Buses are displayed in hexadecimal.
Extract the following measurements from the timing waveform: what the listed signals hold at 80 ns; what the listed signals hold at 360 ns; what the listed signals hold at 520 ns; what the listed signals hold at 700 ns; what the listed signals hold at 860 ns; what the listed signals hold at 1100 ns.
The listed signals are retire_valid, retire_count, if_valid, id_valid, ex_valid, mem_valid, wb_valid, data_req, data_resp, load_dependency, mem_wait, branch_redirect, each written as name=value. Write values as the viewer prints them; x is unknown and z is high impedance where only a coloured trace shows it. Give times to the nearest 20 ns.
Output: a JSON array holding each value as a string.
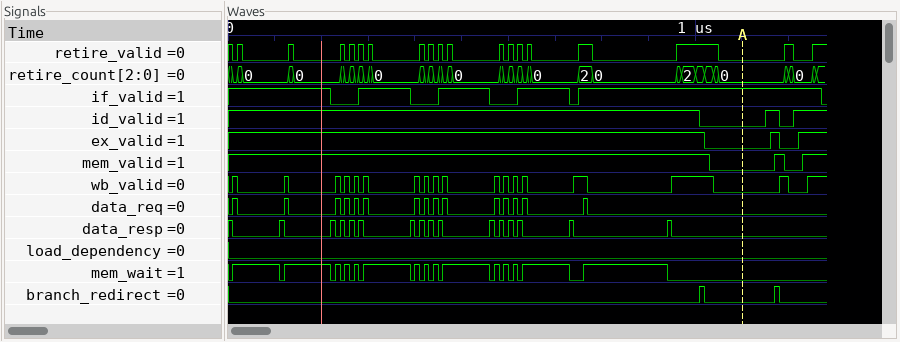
["retire_valid=0, retire_count=0, if_valid=1, id_valid=1, ex_valid=1, mem_valid=1, wb_valid=0, data_req=0, data_resp=0, load_dependency=0, mem_wait=1, branch_redirect=0", "retire_valid=0, retire_count=0, if_valid=1, id_valid=1, ex_valid=1, mem_valid=1, wb_valid=0, data_req=0, data_resp=0, load_dependency=0, mem_wait=1, branch_redirect=0", "retire_valid=0, retire_count=0, if_valid=1, id_valid=1, ex_valid=1, mem_valid=1, wb_valid=0, data_req=0, data_resp=0, load_dependency=0, mem_wait=1, branch_redirect=0", "retire_valid=0, retire_count=0, if_valid=1, id_valid=1, ex_valid=1, mem_valid=1, wb_valid=0, data_req=0, data_resp=0, load_dependency=0, mem_wait=1, branch_redirect=0", "retire_valid=0, retire_count=0, if_valid=1, id_valid=1, ex_valid=1, mem_valid=1, wb_valid=0, data_req=0, data_resp=0, load_dependency=0, mem_wait=1, branch_redirect=0", "retire_valid=0, retire_count=0, if_valid=1, id_valid=0, ex_valid=0, mem_valid=0, wb_valid=0, data_req=0, data_resp=0, load_dependency=0, mem_wait=0, branch_redirect=0"]
